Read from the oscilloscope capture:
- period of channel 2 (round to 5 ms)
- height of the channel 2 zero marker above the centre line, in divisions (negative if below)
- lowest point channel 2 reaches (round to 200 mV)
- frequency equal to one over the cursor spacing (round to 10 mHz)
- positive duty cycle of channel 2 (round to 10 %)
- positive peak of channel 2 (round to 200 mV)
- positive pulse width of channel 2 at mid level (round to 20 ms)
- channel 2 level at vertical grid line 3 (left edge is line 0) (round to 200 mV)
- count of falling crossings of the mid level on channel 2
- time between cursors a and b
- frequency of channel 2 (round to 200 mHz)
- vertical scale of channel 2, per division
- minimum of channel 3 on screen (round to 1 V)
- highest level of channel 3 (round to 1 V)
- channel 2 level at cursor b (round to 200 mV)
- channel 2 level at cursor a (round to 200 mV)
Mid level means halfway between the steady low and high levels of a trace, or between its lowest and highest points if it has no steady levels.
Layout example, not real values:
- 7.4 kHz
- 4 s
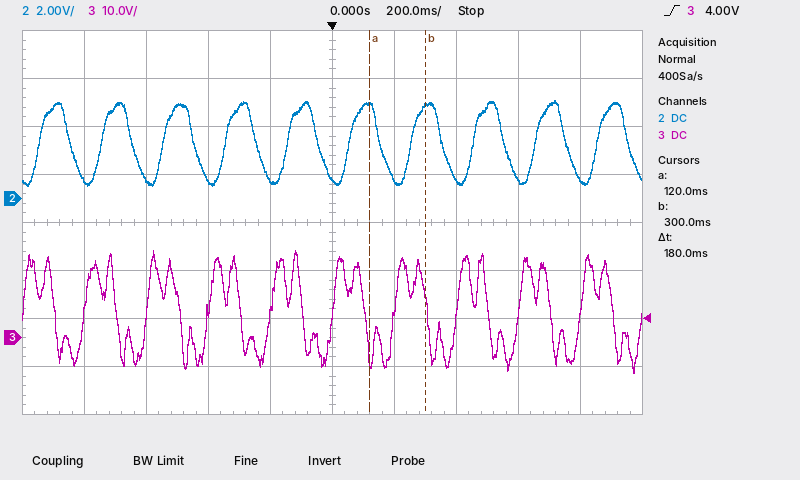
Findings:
- 200 ms
- +0.5 div
- 600 mV
- 5.56 Hz
- 50 %
- 4.0 V
- 100 ms
- 800 mV
- 10
- 180 ms
- 5.0 Hz
- 2 V
- -7 V
- 18 V
- 3.8 V
- 3.8 V
